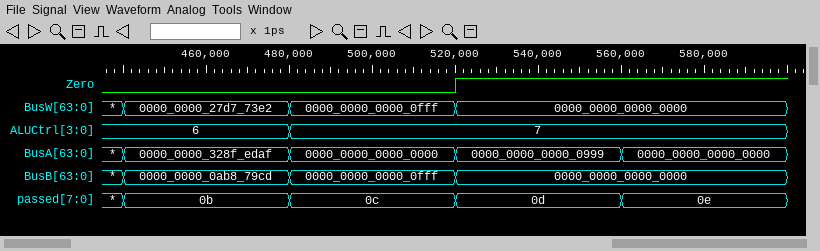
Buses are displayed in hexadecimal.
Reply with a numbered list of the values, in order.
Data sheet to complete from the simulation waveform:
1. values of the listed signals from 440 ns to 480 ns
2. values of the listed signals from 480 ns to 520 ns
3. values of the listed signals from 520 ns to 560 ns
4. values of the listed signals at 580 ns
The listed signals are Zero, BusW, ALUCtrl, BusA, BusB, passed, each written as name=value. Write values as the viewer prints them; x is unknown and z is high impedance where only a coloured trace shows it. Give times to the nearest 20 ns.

1. Zero=0, BusW=0000_0000_27d7_73e2, ALUCtrl=6, BusA=0000_0000_328f_edaf, BusB=0000_0000_0ab8_79cd, passed=0b
2. Zero=0, BusW=0000_0000_0000_0fff, ALUCtrl=7, BusA=0000_0000_0000_0000, BusB=0000_0000_0000_0fff, passed=0c
3. Zero=1, BusW=0000_0000_0000_0000, ALUCtrl=7, BusA=0000_0000_0000_0999, BusB=0000_0000_0000_0000, passed=0d
4. Zero=1, BusW=0000_0000_0000_0000, ALUCtrl=7, BusA=0000_0000_0000_0000, BusB=0000_0000_0000_0000, passed=0e
